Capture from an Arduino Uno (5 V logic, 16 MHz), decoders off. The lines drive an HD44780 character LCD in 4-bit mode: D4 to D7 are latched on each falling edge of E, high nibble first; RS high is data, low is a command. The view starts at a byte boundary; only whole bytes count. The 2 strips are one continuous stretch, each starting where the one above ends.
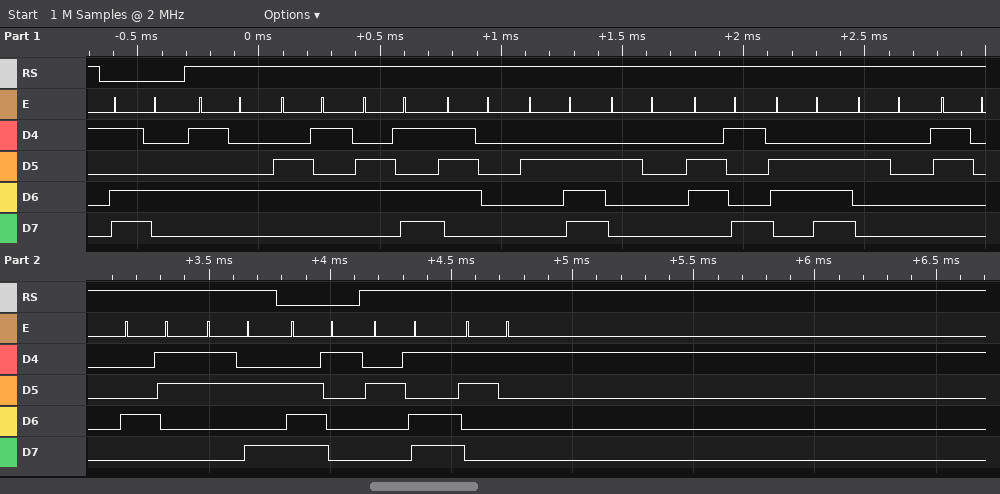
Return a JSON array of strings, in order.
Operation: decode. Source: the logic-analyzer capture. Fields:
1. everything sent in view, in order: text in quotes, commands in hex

["0xD4 \"Temp. in 0C:\" 0xE1 \"-1\""]
